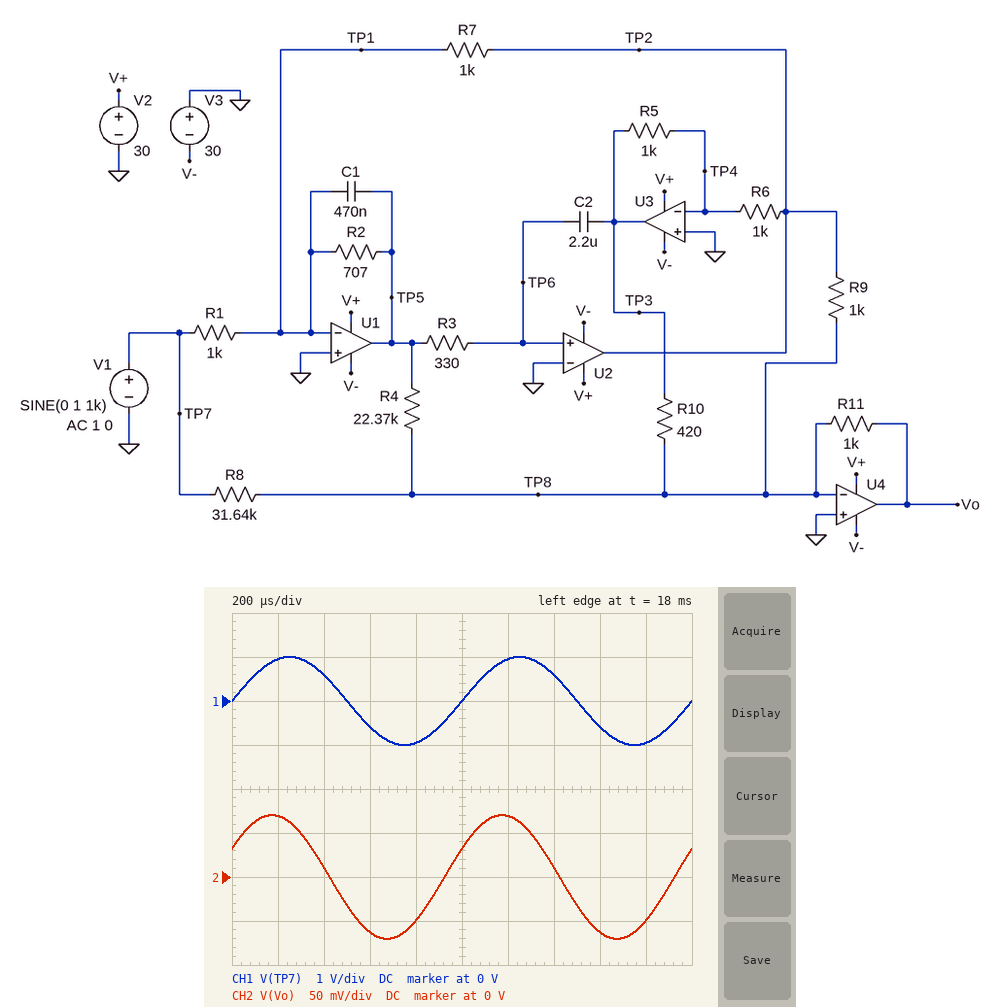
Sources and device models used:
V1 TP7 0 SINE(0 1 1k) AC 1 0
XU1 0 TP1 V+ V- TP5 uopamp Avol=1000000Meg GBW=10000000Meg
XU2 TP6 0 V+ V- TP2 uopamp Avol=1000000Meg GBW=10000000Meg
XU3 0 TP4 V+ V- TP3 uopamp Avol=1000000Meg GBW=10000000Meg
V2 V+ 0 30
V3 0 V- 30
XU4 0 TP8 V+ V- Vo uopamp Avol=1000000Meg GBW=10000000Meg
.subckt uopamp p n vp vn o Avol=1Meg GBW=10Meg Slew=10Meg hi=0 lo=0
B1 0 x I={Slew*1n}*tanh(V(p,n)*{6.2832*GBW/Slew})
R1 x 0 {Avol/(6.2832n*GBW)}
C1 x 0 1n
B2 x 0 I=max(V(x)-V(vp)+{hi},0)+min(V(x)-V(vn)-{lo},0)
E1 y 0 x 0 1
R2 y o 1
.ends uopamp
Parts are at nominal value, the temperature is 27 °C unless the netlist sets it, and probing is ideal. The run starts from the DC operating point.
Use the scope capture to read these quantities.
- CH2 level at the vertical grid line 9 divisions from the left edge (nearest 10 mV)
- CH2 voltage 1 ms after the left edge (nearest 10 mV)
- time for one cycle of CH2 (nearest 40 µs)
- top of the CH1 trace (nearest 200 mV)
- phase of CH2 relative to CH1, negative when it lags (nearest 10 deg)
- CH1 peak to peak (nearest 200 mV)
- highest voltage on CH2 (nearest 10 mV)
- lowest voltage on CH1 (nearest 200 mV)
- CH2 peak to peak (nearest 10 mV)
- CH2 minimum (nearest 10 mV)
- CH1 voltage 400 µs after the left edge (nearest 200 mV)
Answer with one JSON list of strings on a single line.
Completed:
["-50 mV", "30 mV", "1.00 ms", "1.0 V", "30 deg", "2.0 V", "70 mV", "-1.0 V", "140 mV", "-70 mV", "600 mV"]
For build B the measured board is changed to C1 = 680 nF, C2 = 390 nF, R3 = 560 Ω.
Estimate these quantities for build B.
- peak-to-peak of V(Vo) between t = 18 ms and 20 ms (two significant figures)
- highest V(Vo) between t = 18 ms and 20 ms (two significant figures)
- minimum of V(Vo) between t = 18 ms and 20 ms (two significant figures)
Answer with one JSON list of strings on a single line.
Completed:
["470 mV", "230 mV", "-230 mV"]
